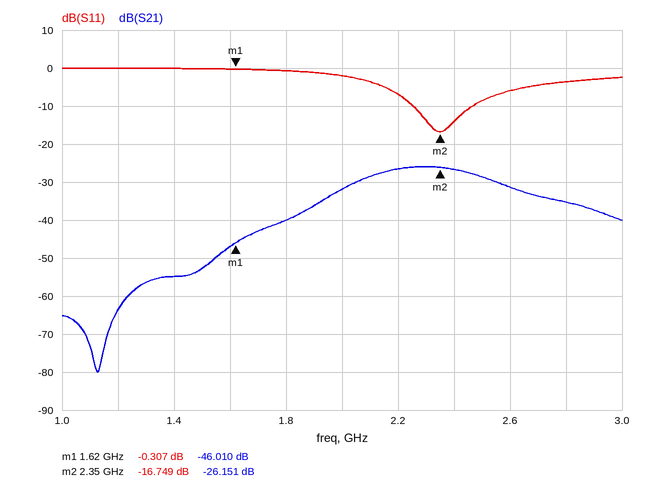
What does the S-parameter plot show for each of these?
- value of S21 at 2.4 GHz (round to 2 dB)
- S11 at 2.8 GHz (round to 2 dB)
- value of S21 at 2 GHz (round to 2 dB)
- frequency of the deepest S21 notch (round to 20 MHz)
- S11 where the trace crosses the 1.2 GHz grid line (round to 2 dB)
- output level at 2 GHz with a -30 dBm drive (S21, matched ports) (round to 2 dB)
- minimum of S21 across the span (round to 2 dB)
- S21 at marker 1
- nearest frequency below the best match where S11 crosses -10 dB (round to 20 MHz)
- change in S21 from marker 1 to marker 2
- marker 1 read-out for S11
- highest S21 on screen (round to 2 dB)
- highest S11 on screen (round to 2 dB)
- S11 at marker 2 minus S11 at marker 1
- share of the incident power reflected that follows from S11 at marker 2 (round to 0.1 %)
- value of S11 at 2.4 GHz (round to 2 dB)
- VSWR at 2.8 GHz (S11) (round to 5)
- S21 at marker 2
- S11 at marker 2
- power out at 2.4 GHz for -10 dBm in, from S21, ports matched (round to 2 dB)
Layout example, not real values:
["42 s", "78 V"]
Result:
["-26 dB", "-4 dB", "-32 dB", "1.12 GHz", "0 dB", "-62 dBm", "-80 dB", "-46.010 dB", "2.26 GHz", "19.859 dB", "-0.307 dB", "-26 dB", "0 dB", "-16.442 dB", "2.1 %", "-14 dB", "5", "-26.151 dB", "-16.749 dB", "-36 dBm"]
